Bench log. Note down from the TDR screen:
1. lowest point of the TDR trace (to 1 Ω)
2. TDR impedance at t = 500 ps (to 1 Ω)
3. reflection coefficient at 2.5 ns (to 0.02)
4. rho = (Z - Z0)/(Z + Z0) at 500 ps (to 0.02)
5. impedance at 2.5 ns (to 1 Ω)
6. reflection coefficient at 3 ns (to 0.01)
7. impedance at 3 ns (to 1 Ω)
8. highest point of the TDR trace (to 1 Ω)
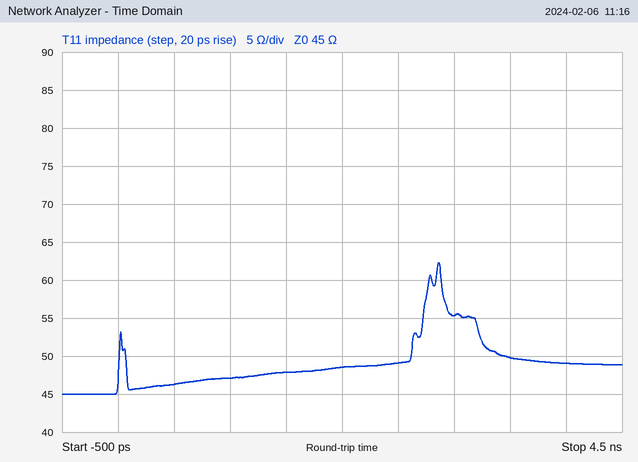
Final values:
45 Ω
46 Ω
+0.04
+0.02
49 Ω
+0.10
55 Ω
62 Ω
